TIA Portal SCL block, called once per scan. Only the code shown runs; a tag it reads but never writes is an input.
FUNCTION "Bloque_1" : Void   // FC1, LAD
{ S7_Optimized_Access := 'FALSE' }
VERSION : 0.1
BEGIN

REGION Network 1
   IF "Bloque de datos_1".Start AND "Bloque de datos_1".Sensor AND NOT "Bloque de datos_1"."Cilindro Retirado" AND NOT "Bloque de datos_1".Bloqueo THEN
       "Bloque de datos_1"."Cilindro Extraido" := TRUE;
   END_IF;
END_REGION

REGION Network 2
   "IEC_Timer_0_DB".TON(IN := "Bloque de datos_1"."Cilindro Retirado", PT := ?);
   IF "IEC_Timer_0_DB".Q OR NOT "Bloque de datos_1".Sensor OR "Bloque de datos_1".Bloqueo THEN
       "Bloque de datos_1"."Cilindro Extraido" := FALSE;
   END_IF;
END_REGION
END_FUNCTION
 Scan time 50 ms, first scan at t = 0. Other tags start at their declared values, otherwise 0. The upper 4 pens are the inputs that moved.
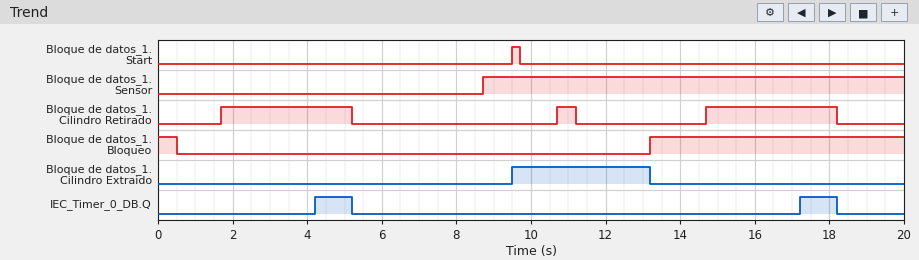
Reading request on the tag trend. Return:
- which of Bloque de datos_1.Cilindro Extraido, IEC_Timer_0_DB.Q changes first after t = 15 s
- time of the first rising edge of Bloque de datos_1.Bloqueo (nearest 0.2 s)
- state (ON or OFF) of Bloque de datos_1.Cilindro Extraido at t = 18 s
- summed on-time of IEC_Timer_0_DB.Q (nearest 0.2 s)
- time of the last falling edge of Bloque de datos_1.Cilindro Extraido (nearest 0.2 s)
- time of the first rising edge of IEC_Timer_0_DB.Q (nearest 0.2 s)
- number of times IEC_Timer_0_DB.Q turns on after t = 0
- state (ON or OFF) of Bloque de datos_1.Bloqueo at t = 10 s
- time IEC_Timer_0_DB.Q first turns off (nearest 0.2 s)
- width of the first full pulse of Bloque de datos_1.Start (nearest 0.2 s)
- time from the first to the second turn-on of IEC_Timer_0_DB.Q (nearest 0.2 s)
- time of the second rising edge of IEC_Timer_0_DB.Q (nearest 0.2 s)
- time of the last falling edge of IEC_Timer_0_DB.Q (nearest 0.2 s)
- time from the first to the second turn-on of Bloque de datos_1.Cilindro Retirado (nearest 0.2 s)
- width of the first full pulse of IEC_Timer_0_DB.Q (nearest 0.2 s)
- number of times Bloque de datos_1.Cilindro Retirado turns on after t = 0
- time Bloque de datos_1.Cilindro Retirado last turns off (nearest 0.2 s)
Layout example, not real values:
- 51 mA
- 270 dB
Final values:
- IEC_Timer_0_DB.Q
- 13.2 s
- OFF
- 2.0 s
- 13.2 s
- 4.2 s
- 2
- OFF
- 5.2 s
- 0.2 s
- 13.0 s
- 17.2 s
- 18.2 s
- 9.0 s
- 1.0 s
- 3
- 18.2 s
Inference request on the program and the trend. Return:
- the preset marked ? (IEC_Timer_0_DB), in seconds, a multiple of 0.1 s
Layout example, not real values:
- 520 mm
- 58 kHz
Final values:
- 2.5 s
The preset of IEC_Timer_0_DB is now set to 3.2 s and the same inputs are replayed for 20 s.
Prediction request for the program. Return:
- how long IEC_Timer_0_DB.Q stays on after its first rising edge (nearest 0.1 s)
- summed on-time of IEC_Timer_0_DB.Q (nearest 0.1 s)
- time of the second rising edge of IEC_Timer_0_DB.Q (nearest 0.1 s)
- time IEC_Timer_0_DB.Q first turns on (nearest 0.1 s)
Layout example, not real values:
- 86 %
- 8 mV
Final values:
- 0.3 s
- 0.6 s
- 17.9 s
- 4.9 s
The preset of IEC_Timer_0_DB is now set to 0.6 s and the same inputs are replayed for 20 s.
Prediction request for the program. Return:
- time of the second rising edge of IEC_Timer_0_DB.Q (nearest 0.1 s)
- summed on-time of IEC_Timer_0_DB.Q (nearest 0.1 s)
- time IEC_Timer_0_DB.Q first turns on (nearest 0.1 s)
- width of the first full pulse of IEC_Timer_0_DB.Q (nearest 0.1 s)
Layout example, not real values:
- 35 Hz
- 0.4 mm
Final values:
- 15.3 s
- 5.8 s
- 2.3 s
- 2.9 s
